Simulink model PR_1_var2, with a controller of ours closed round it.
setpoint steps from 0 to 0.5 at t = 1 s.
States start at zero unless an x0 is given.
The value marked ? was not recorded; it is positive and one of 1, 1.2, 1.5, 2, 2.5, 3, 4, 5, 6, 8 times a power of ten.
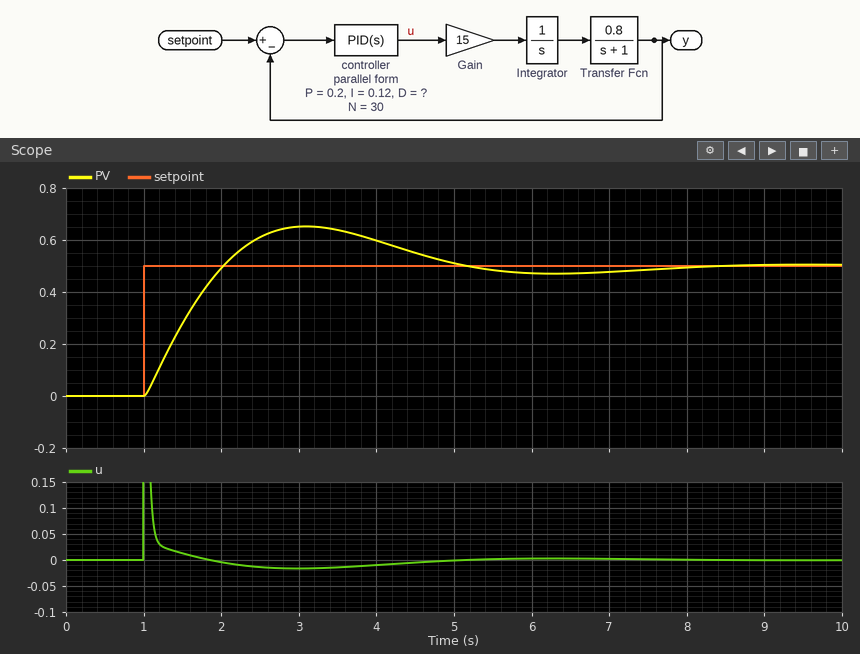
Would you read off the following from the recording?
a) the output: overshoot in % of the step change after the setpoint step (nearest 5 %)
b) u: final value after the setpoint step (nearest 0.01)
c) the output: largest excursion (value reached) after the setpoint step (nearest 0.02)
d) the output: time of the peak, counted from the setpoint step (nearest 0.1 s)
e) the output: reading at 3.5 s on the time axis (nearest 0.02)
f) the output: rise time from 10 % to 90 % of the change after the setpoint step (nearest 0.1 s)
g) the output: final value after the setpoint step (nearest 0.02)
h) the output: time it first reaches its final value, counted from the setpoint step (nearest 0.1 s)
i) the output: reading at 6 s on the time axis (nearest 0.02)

30 %
0.00
0.66
2.1 s
0.64
0.8 s
0.50
1.0 s
0.48
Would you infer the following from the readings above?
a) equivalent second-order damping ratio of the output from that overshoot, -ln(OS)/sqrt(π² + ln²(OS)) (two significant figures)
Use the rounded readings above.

0.36
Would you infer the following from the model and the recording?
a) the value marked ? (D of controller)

0.1
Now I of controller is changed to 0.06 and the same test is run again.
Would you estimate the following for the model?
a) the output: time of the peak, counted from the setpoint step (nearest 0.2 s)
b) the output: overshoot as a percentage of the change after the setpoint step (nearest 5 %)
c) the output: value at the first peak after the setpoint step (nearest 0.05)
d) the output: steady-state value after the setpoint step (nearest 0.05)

2.2 s
20 %
0.60
0.50
